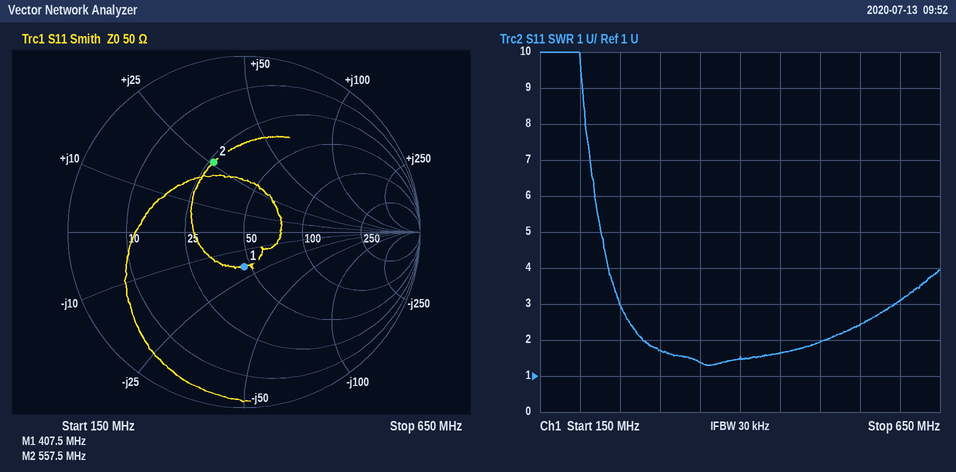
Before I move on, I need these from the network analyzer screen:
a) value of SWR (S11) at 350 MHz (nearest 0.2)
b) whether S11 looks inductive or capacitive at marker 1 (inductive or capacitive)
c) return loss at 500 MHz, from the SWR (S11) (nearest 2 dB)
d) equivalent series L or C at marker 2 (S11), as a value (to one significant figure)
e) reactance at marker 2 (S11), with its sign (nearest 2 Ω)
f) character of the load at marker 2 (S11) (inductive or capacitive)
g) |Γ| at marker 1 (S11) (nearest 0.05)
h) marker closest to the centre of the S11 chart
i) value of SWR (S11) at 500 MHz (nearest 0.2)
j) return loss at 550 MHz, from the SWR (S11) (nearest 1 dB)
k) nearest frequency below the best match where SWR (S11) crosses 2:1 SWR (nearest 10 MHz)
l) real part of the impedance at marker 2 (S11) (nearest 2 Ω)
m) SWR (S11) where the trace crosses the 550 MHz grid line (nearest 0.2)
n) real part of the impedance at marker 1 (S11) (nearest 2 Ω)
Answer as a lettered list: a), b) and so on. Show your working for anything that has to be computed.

a) 1.4
b) capacitive
c) −20 log10((2 − 1)/(2 + 1)) ≈ 10 dB
d) L = 26 Ω/(2π × 557.5 MHz) ≈ 7 nH
e) +26 Ω
f) inductive
g) 0.20
h) marker 1
i) 2.0
j) −20 log10((2.4 − 1)/(2.4 + 1)) ≈ 8 dB
k) 280 MHz
l) 26 Ω
m) 2.4
n) 46 Ω
